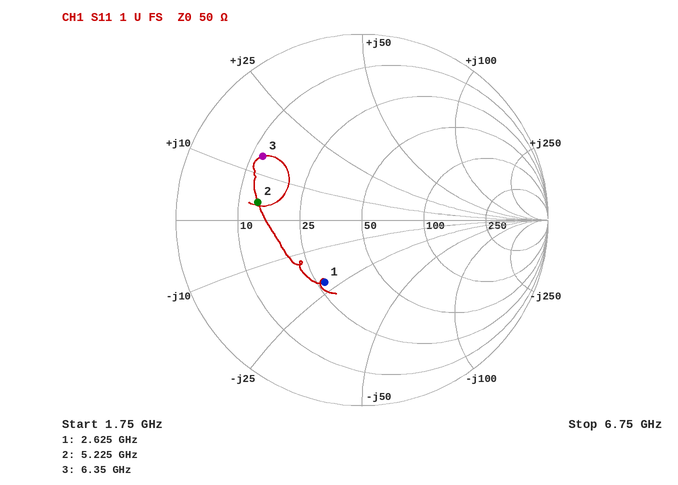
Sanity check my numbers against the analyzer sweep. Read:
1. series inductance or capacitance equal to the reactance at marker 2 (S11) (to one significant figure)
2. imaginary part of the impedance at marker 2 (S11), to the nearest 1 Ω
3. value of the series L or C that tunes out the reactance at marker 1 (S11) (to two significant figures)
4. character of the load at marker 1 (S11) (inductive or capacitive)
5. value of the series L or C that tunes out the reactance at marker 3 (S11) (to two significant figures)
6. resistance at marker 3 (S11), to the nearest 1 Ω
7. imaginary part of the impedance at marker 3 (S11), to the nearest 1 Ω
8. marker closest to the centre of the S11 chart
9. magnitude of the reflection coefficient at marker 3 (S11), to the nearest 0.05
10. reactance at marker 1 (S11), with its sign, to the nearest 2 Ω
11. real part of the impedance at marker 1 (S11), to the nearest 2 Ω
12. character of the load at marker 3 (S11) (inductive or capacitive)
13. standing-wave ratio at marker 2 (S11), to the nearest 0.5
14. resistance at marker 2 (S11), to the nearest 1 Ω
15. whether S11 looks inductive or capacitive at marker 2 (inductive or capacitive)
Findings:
100 pH
+4 Ω
1.3 nH
capacitive
1.8 pF
12 Ω
+14 Ω
marker 1
0.65
-22 Ω
28 Ω
inductive
3.5
14 Ω
inductive
